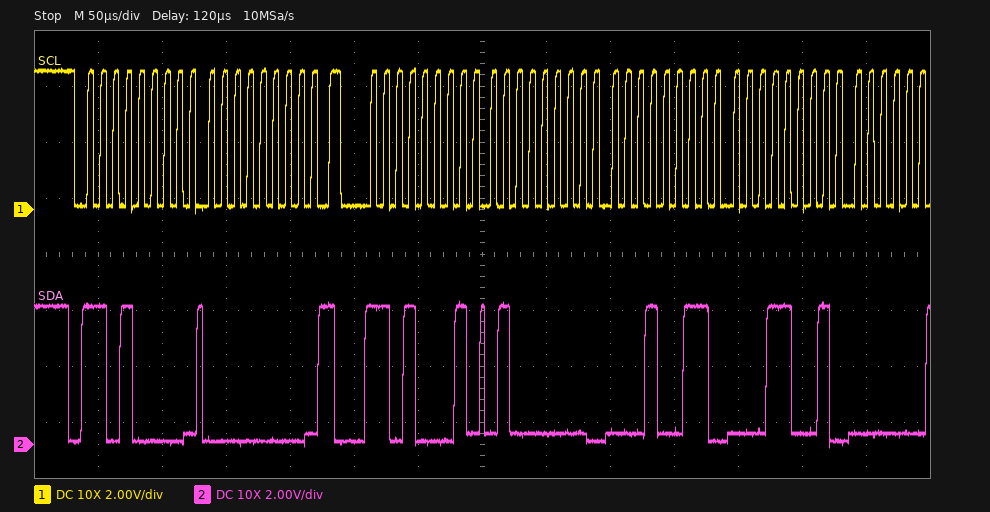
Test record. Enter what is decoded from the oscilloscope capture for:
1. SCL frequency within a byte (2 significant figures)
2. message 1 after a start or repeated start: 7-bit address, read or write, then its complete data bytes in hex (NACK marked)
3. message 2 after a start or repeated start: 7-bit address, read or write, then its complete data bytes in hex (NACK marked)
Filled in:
100 kHz
0x68 write: 00
0x68 read: 40 13 19
